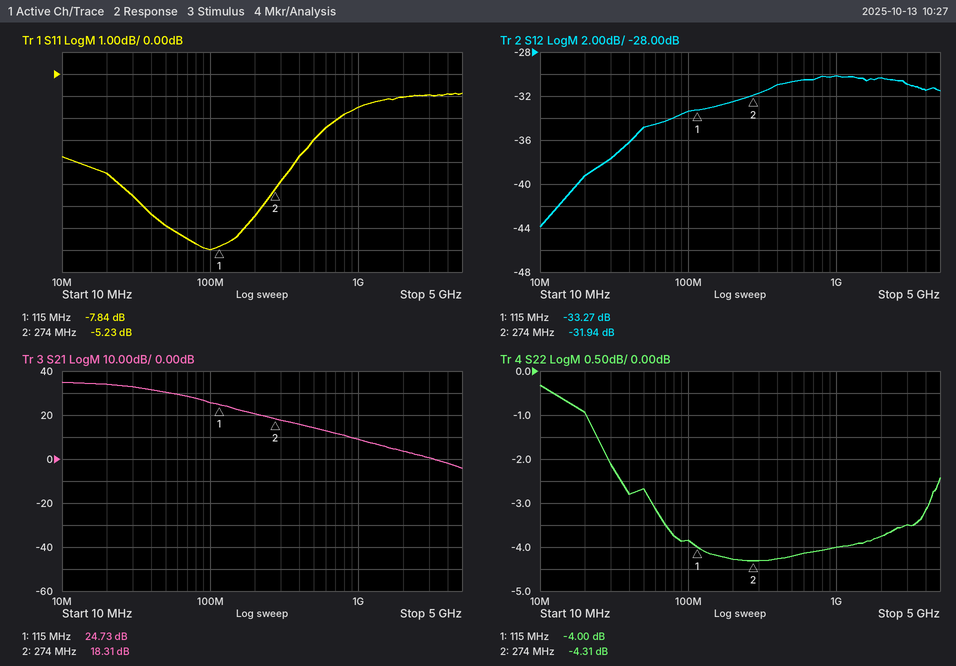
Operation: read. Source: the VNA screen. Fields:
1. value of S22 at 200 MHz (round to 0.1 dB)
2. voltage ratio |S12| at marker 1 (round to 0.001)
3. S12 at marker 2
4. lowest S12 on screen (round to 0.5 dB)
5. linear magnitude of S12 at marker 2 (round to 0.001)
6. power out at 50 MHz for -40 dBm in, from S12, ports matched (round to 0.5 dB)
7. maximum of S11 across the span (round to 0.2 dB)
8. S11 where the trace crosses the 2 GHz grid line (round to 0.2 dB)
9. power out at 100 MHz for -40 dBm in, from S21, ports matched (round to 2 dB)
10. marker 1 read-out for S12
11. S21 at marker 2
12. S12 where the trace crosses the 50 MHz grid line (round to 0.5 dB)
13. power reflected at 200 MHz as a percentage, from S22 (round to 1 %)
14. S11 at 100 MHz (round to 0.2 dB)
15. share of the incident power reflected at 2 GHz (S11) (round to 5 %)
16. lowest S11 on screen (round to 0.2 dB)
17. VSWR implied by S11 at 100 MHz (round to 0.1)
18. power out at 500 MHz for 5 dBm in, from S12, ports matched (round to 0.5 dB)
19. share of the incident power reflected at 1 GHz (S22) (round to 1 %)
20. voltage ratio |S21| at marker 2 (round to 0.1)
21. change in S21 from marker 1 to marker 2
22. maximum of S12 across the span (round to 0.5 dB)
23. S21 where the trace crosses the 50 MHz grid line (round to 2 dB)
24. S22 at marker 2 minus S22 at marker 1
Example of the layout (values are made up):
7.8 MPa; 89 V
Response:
-4.3 dB; 0.022; -31.94 dB; -44.0 dB; 0.025; -75.0 dBm; -0.8 dB; -1.0 dB; -14 dBm; -33.27 dB; 18.31 dB; -35.0 dB; 37 %; -8.0 dB; 80 %; -8.0 dB; 2.3; -25.5 dBm; 40 %; 8.2; -6.42 dB; -30.0 dB; 30 dB; -0.31 dB
